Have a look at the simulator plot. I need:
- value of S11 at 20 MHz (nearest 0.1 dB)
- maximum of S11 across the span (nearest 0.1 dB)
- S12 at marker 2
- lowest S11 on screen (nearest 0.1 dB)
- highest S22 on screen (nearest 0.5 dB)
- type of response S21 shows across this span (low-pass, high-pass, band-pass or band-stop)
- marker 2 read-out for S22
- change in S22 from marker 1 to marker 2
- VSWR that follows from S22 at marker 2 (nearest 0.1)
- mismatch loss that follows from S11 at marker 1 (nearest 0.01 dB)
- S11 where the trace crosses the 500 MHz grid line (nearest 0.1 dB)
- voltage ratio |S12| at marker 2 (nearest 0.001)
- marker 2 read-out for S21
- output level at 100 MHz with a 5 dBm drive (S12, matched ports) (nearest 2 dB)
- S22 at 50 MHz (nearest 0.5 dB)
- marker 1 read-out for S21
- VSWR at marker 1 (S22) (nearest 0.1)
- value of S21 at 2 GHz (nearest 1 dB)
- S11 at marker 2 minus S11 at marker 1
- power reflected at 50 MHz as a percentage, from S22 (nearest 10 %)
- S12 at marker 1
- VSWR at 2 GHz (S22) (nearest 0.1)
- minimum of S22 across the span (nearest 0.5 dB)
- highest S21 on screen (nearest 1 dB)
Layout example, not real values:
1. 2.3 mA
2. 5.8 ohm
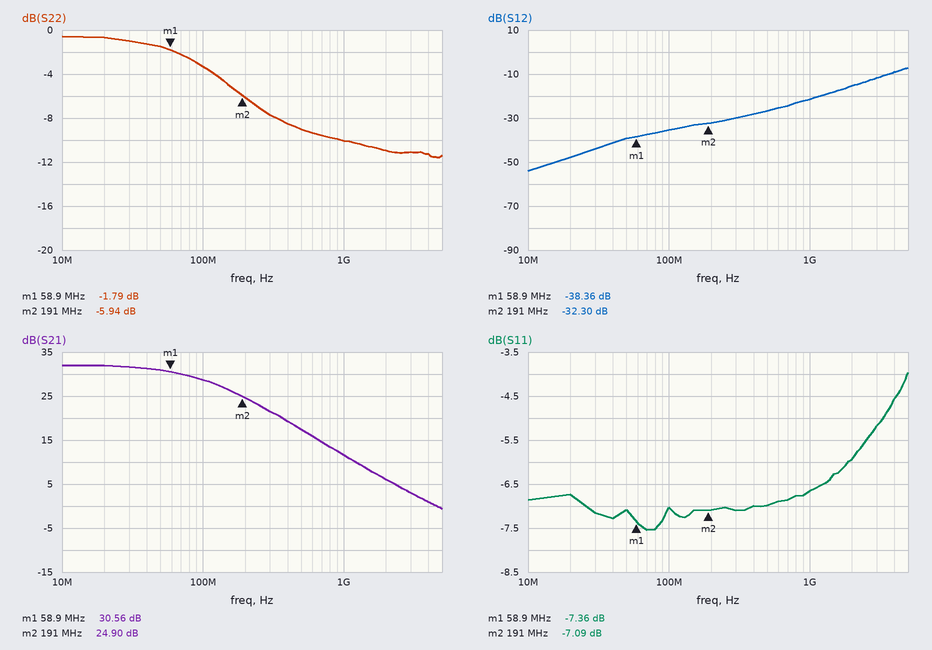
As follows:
1. -6.7 dB
2. -4.0 dB
3. -32.30 dB
4. -7.5 dB
5. -0.5 dB
6. low-pass
7. -5.94 dB
8. -4.15 dB
9. 3.0
10. 0.88 dB
11. -7.0 dB
12. 0.024
13. 24.90 dB
14. -30 dBm
15. -1.5 dB
16. 30.56 dB
17. 9.7
18. 6 dB
19. 0.27 dB
20. 70 %
21. -38.36 dB
22. 1.8
23. -11.5 dB
24. 32 dB
